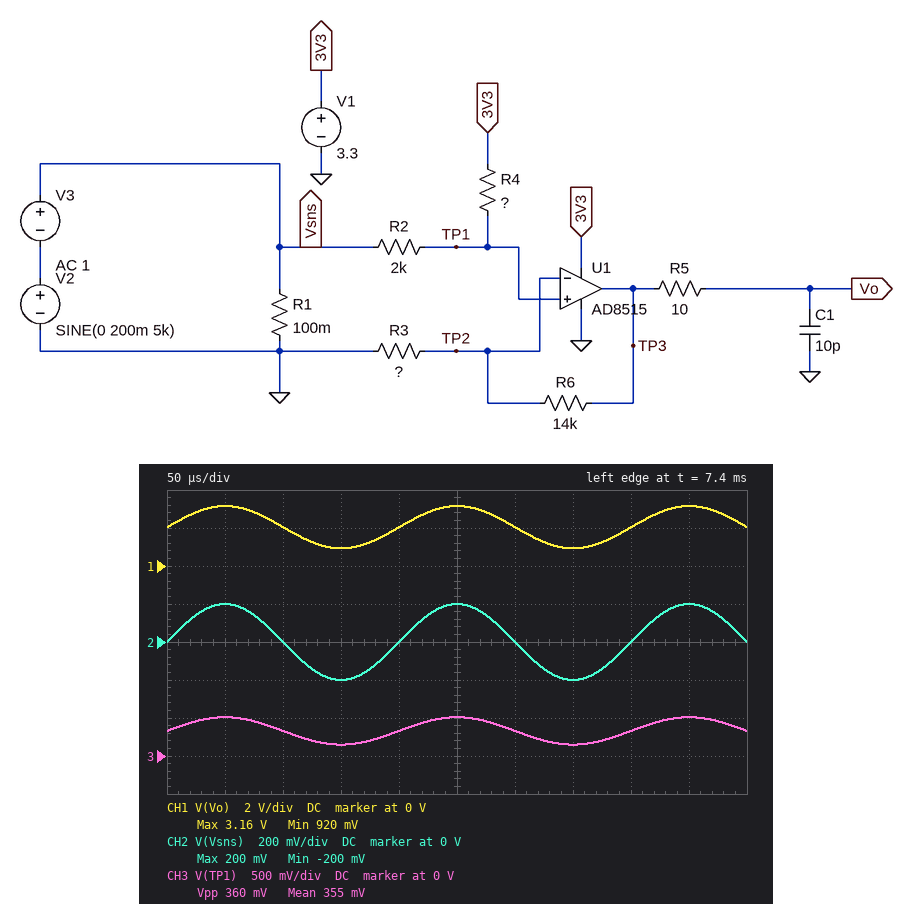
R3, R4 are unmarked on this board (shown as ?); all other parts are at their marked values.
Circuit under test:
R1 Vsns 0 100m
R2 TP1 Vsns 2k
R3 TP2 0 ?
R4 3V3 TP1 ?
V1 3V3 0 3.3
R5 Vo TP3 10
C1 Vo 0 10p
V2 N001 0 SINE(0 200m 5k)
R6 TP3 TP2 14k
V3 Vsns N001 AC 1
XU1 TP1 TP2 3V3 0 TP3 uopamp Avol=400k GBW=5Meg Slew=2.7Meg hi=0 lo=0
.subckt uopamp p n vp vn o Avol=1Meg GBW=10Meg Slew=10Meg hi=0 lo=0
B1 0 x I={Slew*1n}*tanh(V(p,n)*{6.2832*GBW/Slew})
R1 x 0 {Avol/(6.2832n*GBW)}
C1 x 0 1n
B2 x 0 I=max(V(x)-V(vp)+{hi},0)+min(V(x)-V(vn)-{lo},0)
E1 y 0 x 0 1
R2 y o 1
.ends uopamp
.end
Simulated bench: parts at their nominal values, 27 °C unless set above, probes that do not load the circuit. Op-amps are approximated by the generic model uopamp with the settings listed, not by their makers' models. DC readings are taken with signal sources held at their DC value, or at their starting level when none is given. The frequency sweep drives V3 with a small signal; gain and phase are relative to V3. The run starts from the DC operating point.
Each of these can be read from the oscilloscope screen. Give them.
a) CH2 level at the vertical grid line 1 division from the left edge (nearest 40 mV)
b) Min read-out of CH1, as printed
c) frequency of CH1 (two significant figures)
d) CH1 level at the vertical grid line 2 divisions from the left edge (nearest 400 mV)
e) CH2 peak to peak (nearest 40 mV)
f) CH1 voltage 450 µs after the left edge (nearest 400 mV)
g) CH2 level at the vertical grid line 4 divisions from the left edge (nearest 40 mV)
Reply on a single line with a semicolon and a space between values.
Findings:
200 mV; 920 mV; 5.0 kHz; 2.0 V; 400 mV; 3.2 V; 0 V
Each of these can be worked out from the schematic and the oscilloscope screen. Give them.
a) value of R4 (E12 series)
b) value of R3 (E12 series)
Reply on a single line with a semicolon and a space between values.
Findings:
18 kΩ; 2.7 kΩ
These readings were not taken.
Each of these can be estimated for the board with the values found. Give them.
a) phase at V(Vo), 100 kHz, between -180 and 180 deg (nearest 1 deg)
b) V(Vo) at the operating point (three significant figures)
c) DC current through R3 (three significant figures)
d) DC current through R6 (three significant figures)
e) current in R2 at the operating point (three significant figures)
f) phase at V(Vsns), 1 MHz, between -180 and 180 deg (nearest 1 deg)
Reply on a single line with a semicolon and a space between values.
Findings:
-7 deg; 2.04 V; 122 µA; 122 µA; 165 µA; 0 deg
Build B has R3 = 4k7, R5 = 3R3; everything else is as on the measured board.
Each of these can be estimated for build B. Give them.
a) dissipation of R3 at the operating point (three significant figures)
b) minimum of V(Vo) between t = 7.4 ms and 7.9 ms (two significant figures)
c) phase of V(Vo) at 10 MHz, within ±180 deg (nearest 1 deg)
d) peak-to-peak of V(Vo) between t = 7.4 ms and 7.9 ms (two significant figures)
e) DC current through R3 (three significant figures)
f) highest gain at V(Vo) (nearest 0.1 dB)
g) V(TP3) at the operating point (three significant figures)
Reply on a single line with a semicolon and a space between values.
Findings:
23.2 µW; 600 mV; -83 deg; 1.4 V; 70.2 µA; 11.1 dB; 1.31 V
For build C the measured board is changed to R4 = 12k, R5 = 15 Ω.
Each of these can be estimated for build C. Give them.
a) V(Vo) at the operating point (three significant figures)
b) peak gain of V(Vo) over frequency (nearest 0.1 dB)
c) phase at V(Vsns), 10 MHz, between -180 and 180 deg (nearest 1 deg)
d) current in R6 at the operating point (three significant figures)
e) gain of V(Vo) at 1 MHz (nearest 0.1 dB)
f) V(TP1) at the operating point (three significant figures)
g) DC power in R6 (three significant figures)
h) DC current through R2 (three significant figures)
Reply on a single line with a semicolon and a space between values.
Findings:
2.92 V; 14.5 dB; 0 deg; 175 µA; 10.5 dB; 471 mV; 427 µW; 236 µA
